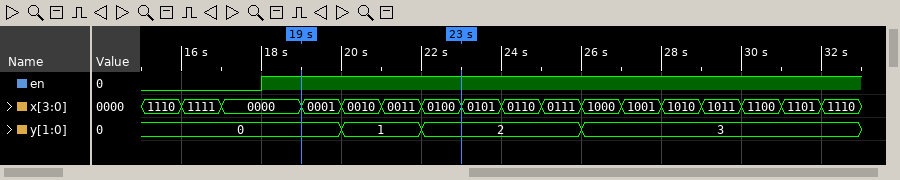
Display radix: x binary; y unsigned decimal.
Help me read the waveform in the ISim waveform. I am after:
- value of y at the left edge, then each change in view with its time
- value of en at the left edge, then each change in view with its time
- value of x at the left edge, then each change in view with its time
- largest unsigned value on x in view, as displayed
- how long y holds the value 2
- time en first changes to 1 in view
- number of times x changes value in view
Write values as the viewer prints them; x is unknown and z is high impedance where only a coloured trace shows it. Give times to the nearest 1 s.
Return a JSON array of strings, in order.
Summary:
["0, 1 at 20 s, 2 at 22 s, 3 at 26 s", "0, 1 at 18 s", "1110, 1111 at 16 s, 0000 at 17 s, 0001 at 19 s, 0010 at 20 s, 0011 at 21 s, 0100 at 22 s, 0101 at 23 s, 0110 at 24 s, 0111 at 25 s, 1000 at 26 s, 1001 at 27 s, 1010 at 28 s, 1011 at 29 s, 1100 at 30 s, 1101 at 31 s, 1110 at 32 s", "1111", "4 s", "18 s", "16"]
